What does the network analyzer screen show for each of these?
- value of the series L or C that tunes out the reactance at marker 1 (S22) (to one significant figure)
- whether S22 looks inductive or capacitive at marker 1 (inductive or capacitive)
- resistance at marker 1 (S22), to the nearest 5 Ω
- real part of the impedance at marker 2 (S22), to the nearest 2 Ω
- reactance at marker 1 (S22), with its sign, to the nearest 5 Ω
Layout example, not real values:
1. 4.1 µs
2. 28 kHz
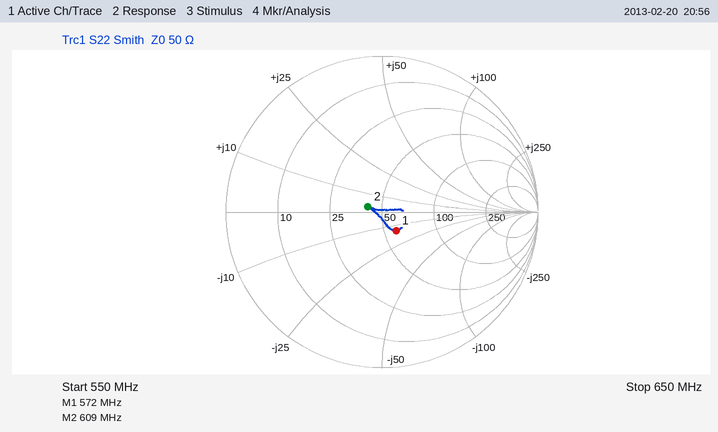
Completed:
1. 4 nH
2. capacitive
3. 60 Ω
4. 42 Ω
5. -15 Ω
